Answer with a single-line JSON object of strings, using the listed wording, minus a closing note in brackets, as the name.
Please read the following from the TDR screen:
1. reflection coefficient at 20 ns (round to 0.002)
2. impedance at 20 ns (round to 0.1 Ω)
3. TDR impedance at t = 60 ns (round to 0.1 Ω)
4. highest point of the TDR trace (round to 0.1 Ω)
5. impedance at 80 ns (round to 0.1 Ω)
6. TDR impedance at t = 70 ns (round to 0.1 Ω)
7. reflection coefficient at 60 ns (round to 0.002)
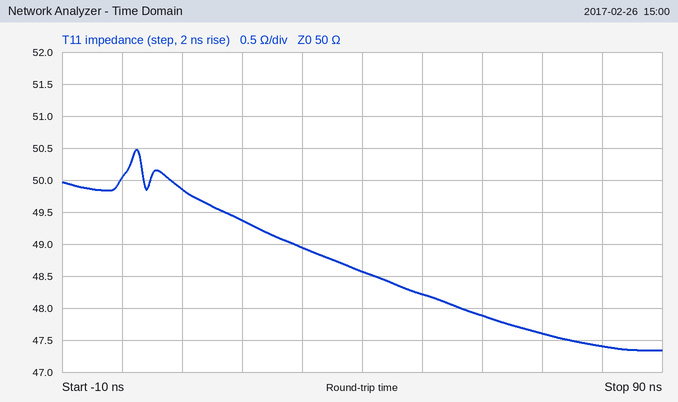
{"reflection coefficient at 20 ns": "-0.006", "impedance at 20 ns": "49.4 Ω", "TDR impedance at t = 60 ns": "47.9 Ω", "highest point of the TDR trace": "50.5 Ω", "impedance at 80 ns": "47.4 Ω", "TDR impedance at t = 70 ns": "47.6 Ω", "reflection coefficient at 60 ns": "-0.022"}
